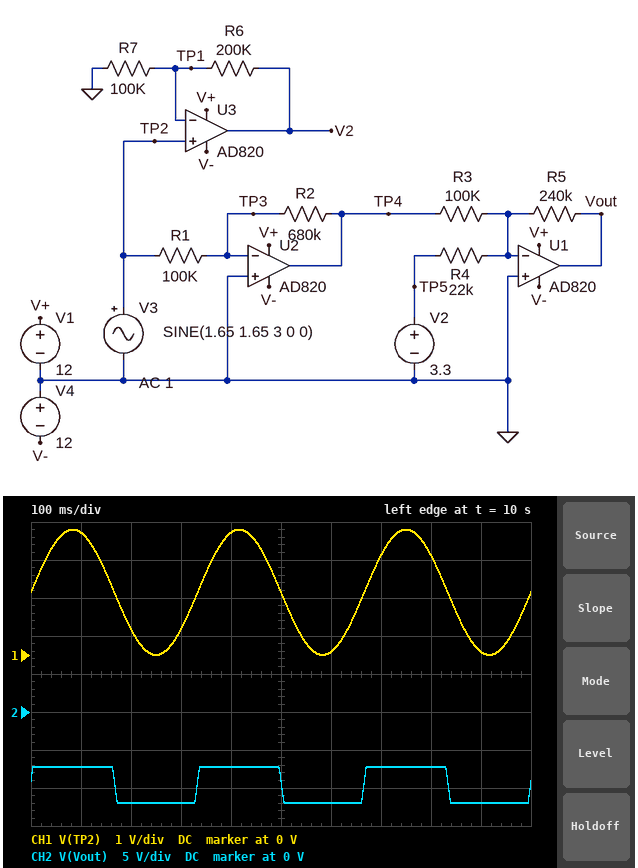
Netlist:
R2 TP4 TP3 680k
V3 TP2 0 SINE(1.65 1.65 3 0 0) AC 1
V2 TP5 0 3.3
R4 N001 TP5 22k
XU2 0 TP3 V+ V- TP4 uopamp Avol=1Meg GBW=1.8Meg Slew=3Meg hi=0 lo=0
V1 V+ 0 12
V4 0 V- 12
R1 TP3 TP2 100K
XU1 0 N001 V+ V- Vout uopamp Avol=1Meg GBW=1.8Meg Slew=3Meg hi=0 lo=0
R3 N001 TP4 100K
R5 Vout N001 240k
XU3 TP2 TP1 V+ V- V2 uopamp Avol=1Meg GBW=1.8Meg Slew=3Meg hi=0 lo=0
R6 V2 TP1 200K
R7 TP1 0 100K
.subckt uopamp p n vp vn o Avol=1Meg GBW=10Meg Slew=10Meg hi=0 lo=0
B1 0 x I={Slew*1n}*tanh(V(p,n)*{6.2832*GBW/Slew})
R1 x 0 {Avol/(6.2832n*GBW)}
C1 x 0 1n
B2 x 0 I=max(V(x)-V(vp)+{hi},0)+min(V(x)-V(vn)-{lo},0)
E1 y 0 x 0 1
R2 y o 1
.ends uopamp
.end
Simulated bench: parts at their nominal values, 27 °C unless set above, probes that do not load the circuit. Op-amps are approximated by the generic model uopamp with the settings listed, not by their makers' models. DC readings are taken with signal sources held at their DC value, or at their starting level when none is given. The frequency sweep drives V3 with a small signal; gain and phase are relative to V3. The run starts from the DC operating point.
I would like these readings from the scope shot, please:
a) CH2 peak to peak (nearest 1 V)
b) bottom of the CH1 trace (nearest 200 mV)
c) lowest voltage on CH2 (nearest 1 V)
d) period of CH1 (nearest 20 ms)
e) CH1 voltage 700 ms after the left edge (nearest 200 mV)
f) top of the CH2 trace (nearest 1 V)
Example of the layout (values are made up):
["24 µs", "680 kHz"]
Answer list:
["5 V", "0 V", "-12 V", "340 ms", "2.6 V", "-7 V"]
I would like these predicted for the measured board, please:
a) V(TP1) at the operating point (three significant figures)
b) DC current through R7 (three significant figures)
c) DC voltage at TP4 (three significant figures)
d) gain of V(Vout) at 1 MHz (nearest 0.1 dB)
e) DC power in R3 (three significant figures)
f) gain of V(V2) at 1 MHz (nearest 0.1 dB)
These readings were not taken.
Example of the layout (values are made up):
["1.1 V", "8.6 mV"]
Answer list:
["1.65 V", "16.5 µA", "-11.2 V", "-6.8 dB", "1.26 mW", "3.8 dB"]
